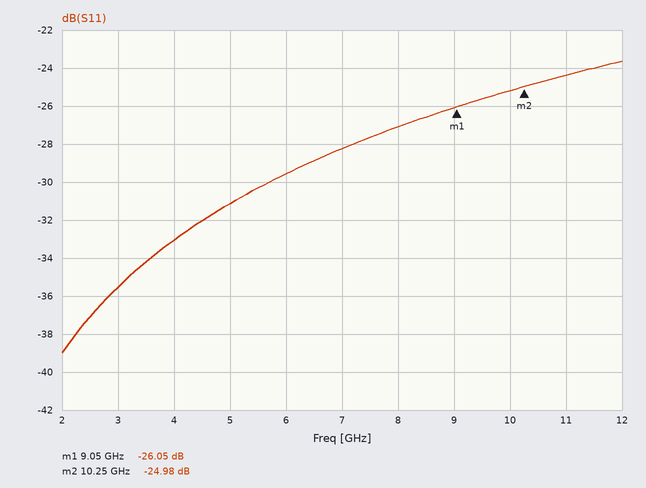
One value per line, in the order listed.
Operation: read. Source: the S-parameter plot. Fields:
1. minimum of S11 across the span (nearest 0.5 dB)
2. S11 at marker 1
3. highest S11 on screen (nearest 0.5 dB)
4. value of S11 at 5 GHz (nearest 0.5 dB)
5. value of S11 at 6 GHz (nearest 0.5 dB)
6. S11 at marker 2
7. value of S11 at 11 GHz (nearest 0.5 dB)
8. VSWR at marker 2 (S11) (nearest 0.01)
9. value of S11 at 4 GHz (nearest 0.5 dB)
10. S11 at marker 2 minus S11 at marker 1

-39.0 dB
-26.05 dB
-23.5 dB
-31.0 dB
-29.5 dB
-24.98 dB
-24.5 dB
1.12
-33.0 dB
1.07 dB
